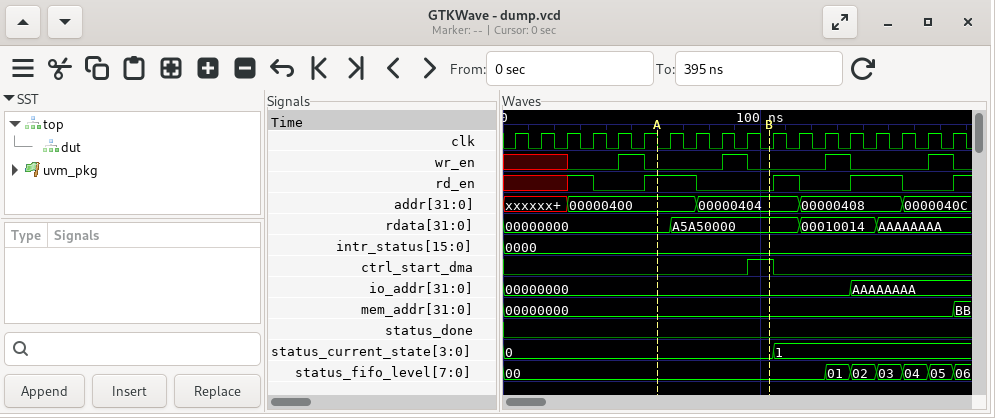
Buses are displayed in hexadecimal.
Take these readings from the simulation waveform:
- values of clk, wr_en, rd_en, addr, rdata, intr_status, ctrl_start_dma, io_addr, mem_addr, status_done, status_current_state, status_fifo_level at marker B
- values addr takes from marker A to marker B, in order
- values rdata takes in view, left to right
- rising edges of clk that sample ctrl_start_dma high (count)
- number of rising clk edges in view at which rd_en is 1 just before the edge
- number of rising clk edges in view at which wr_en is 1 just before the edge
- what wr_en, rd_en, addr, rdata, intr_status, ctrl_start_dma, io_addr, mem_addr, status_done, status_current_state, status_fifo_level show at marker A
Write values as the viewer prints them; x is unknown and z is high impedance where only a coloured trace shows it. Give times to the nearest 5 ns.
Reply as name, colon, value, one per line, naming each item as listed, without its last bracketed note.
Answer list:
values of clk, wr_en, rd_en, addr, rdata, intr_status, ctrl_start_dma, io_addr, mem_addr, status_done, status_current_state, status_fifo_level at marker B: clk=0, wr_en=0, rd_en=0, addr=00000404, rdata=A5A50000, intr_status=0000, ctrl_start_dma=1, io_addr=00000000, mem_addr=00000000, status_done=0, status_current_state=0, status_fifo_level=00
values addr takes from marker A to marker B, in order: 00000400, 00000404
values rdata takes in view, left to right: 00000000, A5A50000, 00010014, AAAAAAAA
rising edges of clk that sample ctrl_start_dma high: 1
number of rising clk edges in view at which rd_en is 1 just before the edge: 6
number of rising clk edges in view at which wr_en is 1 just before the edge: 4
what wr_en, rd_en, addr, rdata, intr_status, ctrl_start_dma, io_addr, mem_addr, status_done, status_current_state, status_fifo_level show at marker A: wr_en=0, rd_en=1, addr=00000400, rdata=00000000, intr_status=0000, ctrl_start_dma=0, io_addr=00000000, mem_addr=00000000, status_done=0, status_current_state=0, status_fifo_level=00
